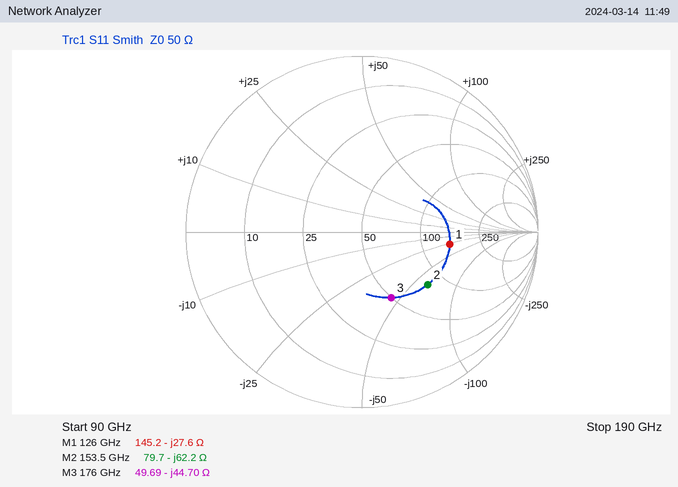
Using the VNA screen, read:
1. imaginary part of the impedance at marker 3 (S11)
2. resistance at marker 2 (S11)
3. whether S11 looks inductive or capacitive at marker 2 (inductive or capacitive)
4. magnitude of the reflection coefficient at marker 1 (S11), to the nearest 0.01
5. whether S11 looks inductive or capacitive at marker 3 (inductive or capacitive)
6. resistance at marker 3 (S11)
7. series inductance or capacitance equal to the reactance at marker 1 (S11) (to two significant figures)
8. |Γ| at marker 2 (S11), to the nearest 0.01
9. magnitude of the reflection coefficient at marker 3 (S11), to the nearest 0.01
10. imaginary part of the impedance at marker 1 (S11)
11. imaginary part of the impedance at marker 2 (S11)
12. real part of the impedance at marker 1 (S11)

-44.70 Ω
79.7 Ω
capacitive
0.50
capacitive
49.69 Ω
46 fF
0.48
0.41
-27.6 Ω
-62.2 Ω
145.2 Ω
